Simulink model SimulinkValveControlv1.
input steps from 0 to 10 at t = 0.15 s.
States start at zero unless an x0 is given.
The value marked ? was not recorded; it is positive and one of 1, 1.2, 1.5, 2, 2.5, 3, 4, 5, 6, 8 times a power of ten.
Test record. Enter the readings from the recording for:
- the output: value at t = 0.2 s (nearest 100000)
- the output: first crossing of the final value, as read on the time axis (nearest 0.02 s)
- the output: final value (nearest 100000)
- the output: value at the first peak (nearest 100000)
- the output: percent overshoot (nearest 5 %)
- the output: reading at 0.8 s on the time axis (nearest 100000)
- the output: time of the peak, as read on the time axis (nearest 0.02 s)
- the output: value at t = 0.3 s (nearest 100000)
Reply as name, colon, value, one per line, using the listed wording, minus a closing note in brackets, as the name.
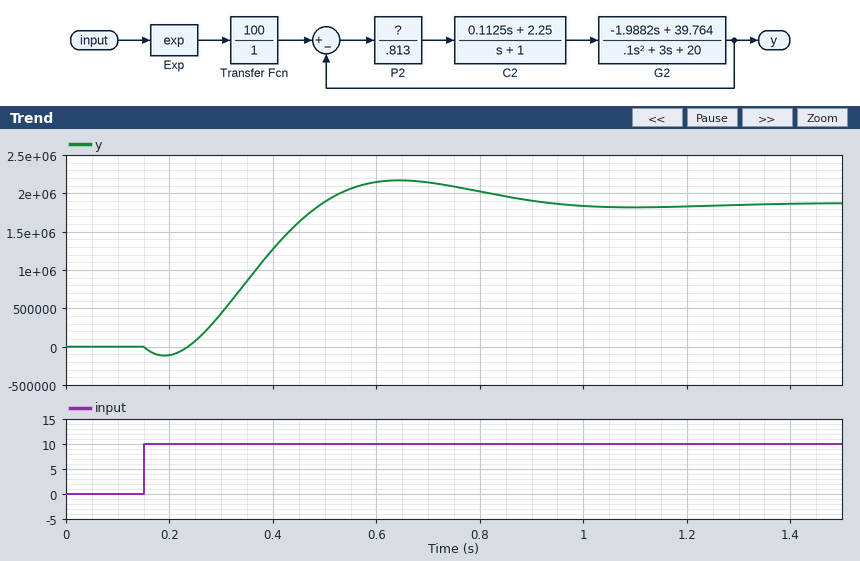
the output: value at t = 0.2 s: -100000
the output: first crossing of the final value, as read on the time axis: 0.50 s
the output: final value: 1900000
the output: value at the first peak: 2200000
the output: percent overshoot: 15 %
the output: reading at 0.8 s on the time axis: 2000000
the output: time of the peak, as read on the time axis: 0.64 s
the output: value at t = 0.3 s: 400000
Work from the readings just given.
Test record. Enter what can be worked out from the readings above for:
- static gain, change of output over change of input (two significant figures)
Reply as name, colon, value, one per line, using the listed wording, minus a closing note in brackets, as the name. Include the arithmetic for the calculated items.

static gain, change of output over change of input: (1.9e+06 - 0) / (10 - 0) = 190000
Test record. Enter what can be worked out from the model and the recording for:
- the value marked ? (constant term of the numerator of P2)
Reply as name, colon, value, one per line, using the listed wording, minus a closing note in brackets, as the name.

the value marked ?: 1
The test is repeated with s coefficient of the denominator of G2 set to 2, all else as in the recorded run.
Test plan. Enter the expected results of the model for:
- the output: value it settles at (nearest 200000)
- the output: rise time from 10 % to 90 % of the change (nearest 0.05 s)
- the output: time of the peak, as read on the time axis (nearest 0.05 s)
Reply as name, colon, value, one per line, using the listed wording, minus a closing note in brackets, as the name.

the output: value it settles at: 1800000
the output: rise time from 10 % to 90 % of the change: 0.15 s
the output: time of the peak, as read on the time axis: 0.55 s
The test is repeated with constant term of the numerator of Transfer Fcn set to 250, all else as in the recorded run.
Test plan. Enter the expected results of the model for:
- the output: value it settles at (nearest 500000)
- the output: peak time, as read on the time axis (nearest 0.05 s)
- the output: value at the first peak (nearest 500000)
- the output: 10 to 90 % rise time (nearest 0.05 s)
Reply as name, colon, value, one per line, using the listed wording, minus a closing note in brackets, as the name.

the output: value it settles at: 4500000
the output: peak time, as read on the time axis: 0.65 s
the output: value at the first peak: 5500000
the output: 10 to 90 % rise time: 0.20 s
